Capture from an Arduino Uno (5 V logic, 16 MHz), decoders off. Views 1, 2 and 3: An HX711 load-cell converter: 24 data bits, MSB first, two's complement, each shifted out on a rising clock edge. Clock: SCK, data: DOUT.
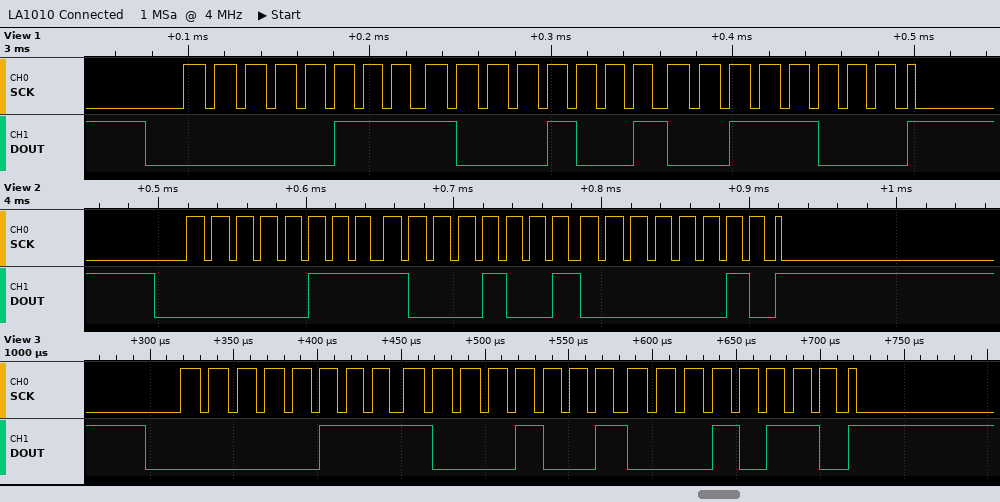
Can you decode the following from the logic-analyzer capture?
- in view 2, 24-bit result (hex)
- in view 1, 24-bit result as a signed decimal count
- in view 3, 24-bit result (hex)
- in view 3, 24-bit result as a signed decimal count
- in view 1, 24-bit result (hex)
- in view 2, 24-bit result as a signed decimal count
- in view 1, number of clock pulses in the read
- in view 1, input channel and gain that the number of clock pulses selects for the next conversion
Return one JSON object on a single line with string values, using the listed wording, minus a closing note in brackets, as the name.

{"in view 2, 24-bit result": "0x078902", "in view 1, 24-bit result as a signed decimal count": "493880", "in view 3, 24-bit result": "0x078916", "in view 3, 24-bit result as a signed decimal count": "493846", "in view 1, 24-bit result": "0x078938", "in view 2, 24-bit result as a signed decimal count": "493826", "in view 1, number of clock pulses in the read": "25", "in view 1, input channel and gain that the number of clock pulses selects for the next conversion": "channel A, gain 128"}
